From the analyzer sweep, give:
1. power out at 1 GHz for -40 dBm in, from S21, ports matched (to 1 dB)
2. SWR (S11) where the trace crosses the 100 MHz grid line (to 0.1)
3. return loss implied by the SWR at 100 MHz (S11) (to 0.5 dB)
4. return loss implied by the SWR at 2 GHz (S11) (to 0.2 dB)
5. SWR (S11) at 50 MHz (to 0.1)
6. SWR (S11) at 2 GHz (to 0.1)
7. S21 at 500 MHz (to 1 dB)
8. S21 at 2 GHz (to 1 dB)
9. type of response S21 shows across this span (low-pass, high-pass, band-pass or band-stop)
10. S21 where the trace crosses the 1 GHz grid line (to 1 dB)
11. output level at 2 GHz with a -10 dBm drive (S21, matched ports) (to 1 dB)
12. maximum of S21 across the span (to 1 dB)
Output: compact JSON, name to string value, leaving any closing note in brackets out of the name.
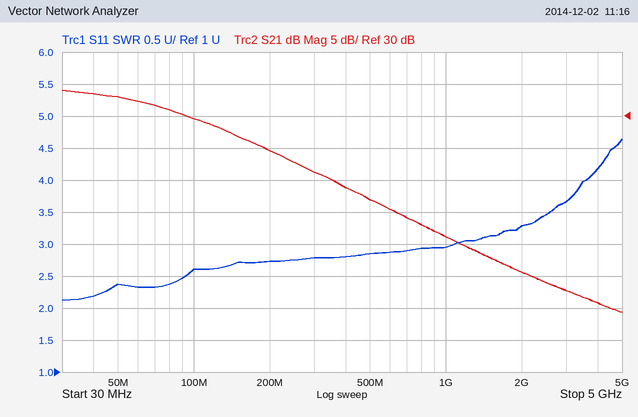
{"power out at 1 GHz for -40 dBm in, from S21, ports matched": "-29 dBm", "SWR (S11) where the trace crosses the 100 MHz grid line": "2.6", "return loss implied by the SWR at 100 MHz (S11)": "7.0 dB", "return loss implied by the SWR at 2 GHz (S11)": "5.4 dB", "SWR (S11) at 50 MHz": "2.4", "SWR (S11) at 2 GHz": "3.3", "S21 at 500 MHz": "17 dB", "S21 at 2 GHz": "6 dB", "type of response S21 shows across this span": "low-pass", "S21 where the trace crosses the 1 GHz grid line": "11 dB", "output level at 2 GHz with a -10 dBm drive (S21, matched ports)": "-4 dBm", "maximum of S21 across the span": "34 dB"}
